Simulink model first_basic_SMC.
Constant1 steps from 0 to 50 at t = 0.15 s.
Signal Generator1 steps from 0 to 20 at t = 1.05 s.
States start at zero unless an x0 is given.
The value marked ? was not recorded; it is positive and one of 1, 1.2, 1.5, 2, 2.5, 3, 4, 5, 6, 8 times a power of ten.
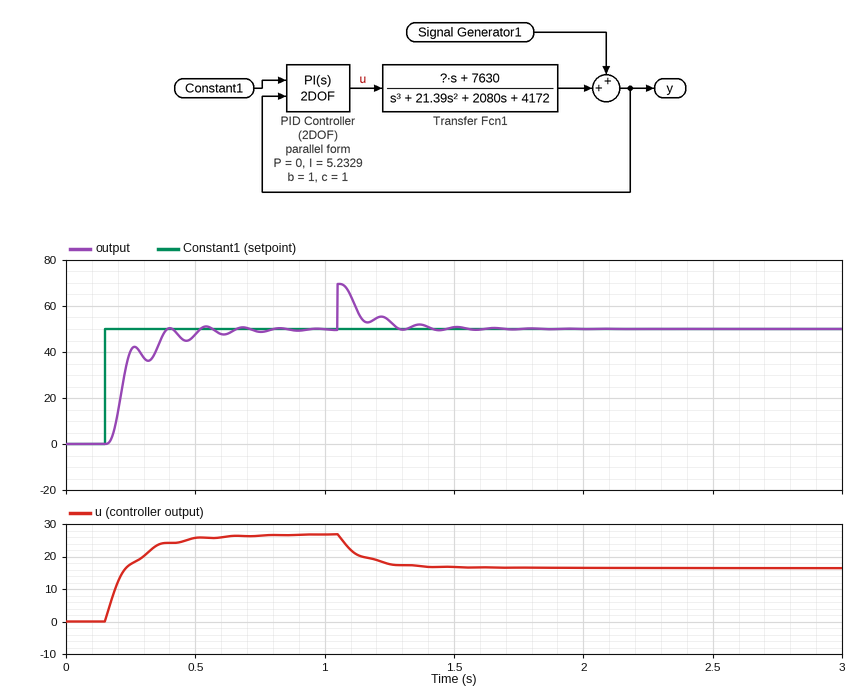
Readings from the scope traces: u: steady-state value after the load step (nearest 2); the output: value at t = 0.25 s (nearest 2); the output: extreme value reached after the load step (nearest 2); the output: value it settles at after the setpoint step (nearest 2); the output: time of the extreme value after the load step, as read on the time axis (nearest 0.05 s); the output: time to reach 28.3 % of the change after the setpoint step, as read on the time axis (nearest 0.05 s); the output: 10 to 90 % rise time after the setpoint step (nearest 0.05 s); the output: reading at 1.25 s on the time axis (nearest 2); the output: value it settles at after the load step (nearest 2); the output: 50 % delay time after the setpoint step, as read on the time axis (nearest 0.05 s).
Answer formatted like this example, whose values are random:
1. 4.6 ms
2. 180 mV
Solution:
1. 16
2. 40
3. 70
4. 50
5. 1.05 s
6. 0.20 s
7. 0.20 s
8. 54
9. 50
10. 0.20 s
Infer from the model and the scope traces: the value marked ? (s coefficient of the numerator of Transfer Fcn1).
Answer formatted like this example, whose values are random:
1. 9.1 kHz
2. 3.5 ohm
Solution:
1. 4000
